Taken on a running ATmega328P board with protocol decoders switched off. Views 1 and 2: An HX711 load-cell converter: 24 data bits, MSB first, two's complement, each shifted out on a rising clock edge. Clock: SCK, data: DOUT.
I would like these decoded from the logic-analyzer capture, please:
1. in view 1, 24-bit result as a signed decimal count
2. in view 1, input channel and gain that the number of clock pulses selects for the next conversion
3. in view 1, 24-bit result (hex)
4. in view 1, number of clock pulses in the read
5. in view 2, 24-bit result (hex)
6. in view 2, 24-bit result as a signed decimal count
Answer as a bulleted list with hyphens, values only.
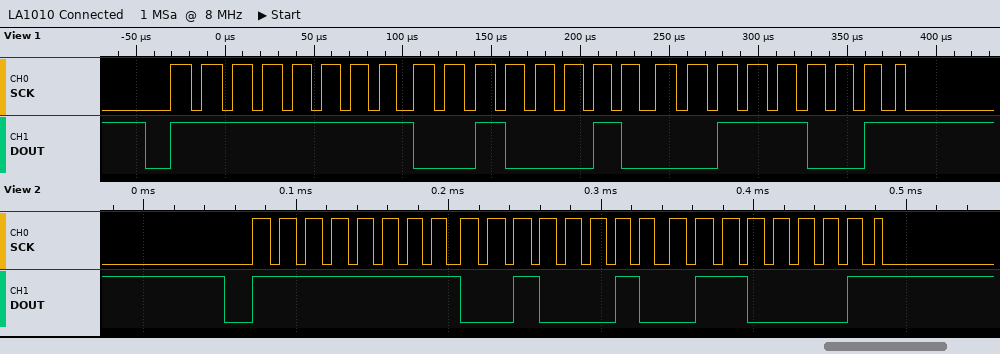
- -56775
- channel A, gain 128
- 0xFF2239
- 25
- 0xFF2261
- -56735
